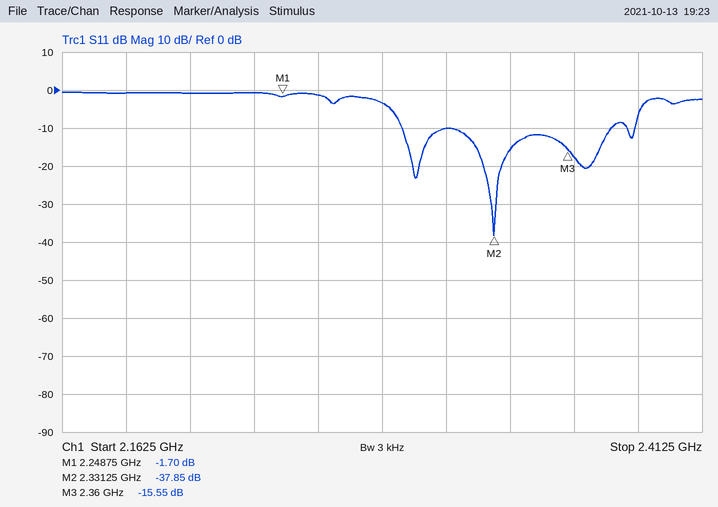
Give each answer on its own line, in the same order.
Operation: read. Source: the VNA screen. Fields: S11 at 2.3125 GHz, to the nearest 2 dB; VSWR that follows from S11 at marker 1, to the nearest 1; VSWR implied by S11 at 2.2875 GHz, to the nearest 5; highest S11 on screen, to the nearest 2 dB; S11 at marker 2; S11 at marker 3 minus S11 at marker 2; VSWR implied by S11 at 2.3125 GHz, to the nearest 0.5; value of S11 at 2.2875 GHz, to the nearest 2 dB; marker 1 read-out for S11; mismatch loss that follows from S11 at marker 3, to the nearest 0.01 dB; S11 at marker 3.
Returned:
-10 dB
10
5
0 dB
-37.85 dB
22.30 dB
2.0
-4 dB
-1.70 dB
0.12 dB
-15.55 dB
